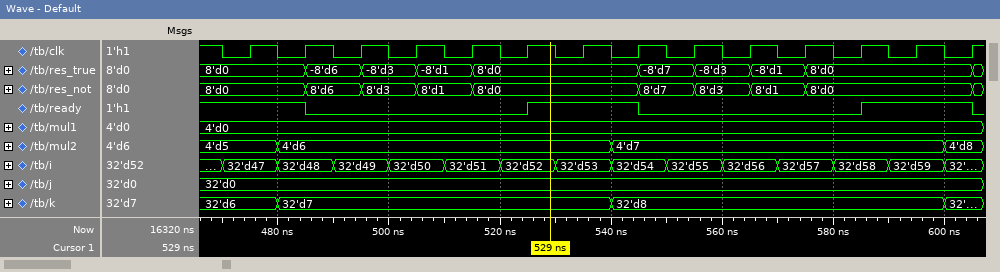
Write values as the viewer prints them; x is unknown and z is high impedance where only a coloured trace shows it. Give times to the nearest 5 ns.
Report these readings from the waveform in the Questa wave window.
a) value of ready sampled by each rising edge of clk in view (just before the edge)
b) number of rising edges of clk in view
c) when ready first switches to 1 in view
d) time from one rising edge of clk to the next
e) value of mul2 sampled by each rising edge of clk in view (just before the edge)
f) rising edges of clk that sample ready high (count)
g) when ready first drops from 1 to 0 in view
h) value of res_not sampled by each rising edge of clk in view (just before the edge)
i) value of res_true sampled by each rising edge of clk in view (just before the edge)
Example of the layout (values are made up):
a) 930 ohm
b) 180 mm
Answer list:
a) 1 1 0 0 0 0 1 1 0 0 0 0 1 1
b) 14
c) 525 ns
d) 10 ns
e) 4'd5, 4'd6, 4'd6, 4'd6, 4'd6, 4'd6, 4'd6, 4'd7, 4'd7, 4'd7, 4'd7, 4'd7, 4'd7, 4'd8
f) 6
g) 485 ns
h) 8'd0, 8'd0, 8'd6, 8'd3, 8'd1, 8'd0, 8'd0, 8'd0, 8'd7, 8'd3, 8'd1, 8'd0, 8'd0, 8'd0
i) 8'd0, 8'd0, -8'd6, -8'd3, -8'd1, 8'd0, 8'd0, 8'd0, -8'd7, -8'd3, -8'd1, 8'd0, 8'd0, 8'd0
